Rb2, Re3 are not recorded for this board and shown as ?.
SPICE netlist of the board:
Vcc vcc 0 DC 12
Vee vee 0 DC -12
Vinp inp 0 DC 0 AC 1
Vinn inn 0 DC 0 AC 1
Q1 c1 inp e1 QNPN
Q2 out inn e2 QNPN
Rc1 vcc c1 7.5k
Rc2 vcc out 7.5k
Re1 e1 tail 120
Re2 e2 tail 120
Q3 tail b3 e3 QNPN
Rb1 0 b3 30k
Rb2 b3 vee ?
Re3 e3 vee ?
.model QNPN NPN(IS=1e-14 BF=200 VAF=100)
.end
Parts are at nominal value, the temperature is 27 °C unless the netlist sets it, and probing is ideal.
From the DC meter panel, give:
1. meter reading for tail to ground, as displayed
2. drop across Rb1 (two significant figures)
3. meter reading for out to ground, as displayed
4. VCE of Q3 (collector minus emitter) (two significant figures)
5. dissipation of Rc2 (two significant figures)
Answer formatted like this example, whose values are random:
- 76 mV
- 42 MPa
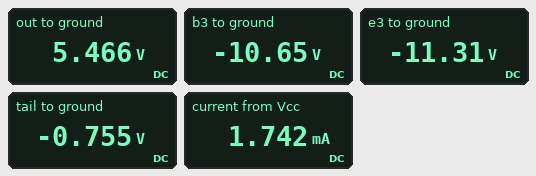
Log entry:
- -0.755 V
- 11 V
- 5.466 V
- 11 V
- 5.7 mW
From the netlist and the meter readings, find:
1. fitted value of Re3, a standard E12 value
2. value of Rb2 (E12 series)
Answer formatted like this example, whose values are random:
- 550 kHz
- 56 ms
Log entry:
- 390 Ω
- 3.9 kΩ
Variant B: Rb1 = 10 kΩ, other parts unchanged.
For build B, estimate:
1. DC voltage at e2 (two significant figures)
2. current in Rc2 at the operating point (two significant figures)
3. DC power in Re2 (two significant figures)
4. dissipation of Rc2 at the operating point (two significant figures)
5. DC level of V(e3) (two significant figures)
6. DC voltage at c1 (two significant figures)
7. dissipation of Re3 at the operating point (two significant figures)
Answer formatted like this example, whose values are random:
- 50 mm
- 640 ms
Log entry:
- -700 mV
- 1.7 mA
- 1.3 mW
- 21 mW
- -9.4 V
- -670 mV
- 17 mW
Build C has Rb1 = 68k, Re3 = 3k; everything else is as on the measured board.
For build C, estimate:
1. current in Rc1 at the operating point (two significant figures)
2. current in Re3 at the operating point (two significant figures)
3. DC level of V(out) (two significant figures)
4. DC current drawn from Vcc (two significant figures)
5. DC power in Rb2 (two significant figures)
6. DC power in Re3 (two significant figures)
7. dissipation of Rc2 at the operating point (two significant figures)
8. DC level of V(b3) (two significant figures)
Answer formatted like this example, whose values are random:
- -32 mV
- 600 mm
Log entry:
- 15 µA
- 30 µA
- 12 V
- 29 µA
- 110 µW
- 2.6 µW
- 1.6 µW
- -11 V
